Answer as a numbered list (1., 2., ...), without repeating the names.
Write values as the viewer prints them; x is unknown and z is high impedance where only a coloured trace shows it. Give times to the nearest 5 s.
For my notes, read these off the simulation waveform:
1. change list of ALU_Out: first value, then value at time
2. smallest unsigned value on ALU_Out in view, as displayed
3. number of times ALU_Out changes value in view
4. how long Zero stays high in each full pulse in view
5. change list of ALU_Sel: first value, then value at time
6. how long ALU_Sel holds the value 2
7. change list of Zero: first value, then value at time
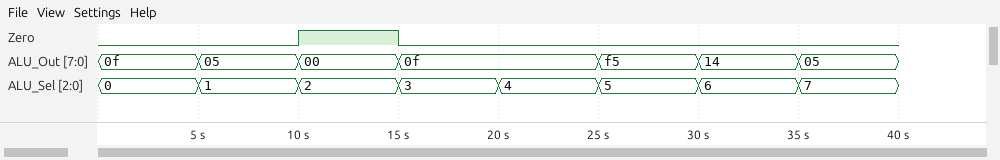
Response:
1. 0f, 05 at 5 s, 00 at 10 s, 0f at 15 s, f5 at 25 s, 14 at 30 s, 05 at 35 s
2. 00
3. 6
4. 5 s
5. 0, 1 at 5 s, 2 at 10 s, 3 at 15 s, 4 at 20 s, 5 at 25 s, 6 at 30 s, 7 at 35 s
6. 5 s
7. 0, 1 at 10 s, 0 at 15 s
